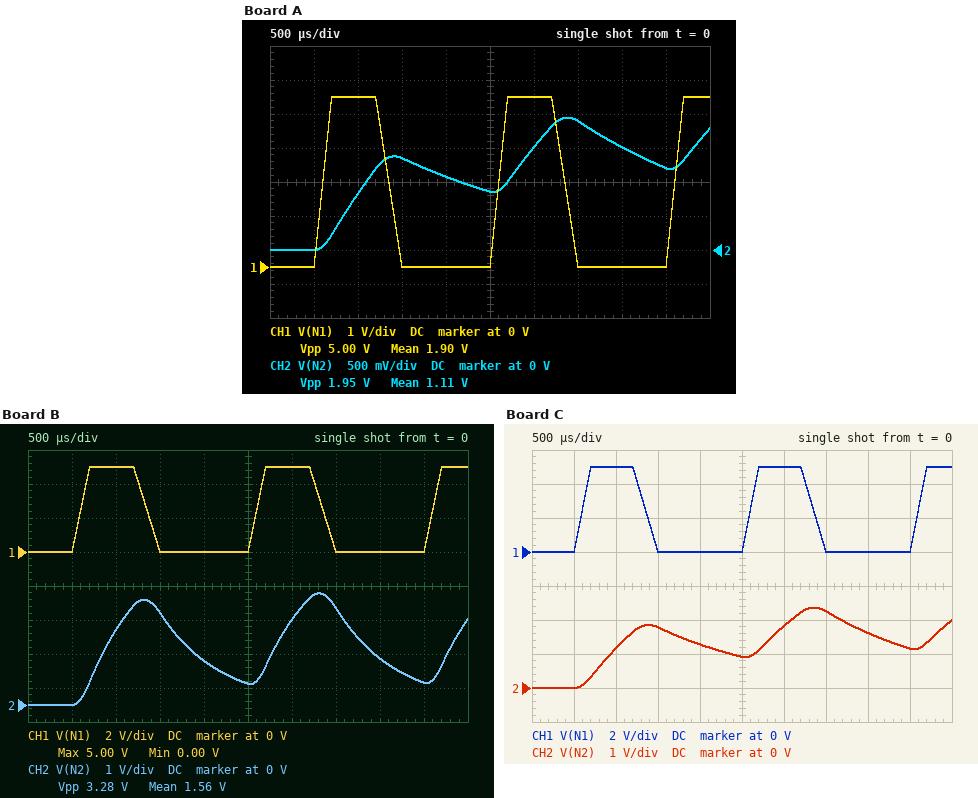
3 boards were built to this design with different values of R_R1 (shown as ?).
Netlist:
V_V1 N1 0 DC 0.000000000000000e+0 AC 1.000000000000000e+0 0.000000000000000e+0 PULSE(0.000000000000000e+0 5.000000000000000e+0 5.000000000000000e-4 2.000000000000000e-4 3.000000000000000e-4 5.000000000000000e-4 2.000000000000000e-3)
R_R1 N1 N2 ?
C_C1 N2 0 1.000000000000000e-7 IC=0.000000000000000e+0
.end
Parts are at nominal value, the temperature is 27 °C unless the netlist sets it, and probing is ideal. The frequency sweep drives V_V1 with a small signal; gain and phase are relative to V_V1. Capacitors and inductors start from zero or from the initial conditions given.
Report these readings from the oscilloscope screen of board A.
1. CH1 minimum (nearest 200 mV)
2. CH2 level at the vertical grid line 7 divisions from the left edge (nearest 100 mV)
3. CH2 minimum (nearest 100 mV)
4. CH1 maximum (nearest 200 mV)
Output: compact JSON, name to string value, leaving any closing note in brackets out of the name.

{"CH1 minimum": "0 V", "CH2 level at the vertical grid line 7 divisions from the left edge": "1.9 V", "CH2 minimum": "0 V", "CH1 maximum": "5.0 V"}
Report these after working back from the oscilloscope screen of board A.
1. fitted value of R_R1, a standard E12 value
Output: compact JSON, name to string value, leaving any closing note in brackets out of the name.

{"fitted value of R_R1, a standard E12 value": "22 kΩ"}
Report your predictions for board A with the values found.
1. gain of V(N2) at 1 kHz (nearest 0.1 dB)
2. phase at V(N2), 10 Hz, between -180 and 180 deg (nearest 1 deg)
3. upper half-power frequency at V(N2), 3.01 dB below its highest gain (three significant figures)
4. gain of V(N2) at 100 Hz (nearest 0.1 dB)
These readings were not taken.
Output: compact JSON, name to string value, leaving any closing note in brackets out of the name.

{"gain of V(N2) at 1 kHz": "-22.8 dB", "phase at V(N2), 10 Hz, between -180 and 180 deg": "-8 deg", "upper half-power frequency at V(N2), 3.01 dB below its highest gain": "72.3 Hz", "gain of V(N2) at 100 Hz": "-4.6 dB"}
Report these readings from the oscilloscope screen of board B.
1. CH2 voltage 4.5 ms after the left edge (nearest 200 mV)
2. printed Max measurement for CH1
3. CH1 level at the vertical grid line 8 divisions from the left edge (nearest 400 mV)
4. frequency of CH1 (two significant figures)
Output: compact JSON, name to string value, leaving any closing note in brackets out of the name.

{"CH2 voltage 4.5 ms after the left edge": "600 mV", "printed Max measurement for CH1": "5.00 V", "CH1 level at the vertical grid line 8 divisions from the left edge": "0 V", "frequency of CH1": "500 Hz"}
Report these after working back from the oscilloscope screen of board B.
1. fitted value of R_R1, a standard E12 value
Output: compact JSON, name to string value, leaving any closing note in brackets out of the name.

{"fitted value of R_R1, a standard E12 value": "6.8 kΩ"}
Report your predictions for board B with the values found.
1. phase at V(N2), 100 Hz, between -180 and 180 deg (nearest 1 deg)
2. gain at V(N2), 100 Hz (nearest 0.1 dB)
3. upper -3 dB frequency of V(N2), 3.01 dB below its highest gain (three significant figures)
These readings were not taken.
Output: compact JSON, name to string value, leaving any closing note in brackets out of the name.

{"phase at V(N2), 100 Hz, between -180 and 180 deg": "-23 deg", "gain at V(N2), 100 Hz": "-0.7 dB", "upper -3 dB frequency of V(N2), 3.01 dB below its highest gain": "234 Hz"}
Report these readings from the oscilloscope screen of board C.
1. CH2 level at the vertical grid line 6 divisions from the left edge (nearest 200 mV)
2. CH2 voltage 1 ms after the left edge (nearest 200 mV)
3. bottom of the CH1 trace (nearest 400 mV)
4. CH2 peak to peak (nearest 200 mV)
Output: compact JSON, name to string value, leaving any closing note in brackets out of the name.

{"CH2 level at the vertical grid line 6 divisions from the left edge": "1.8 V", "CH2 voltage 1 ms after the left edge": "1.2 V", "bottom of the CH1 trace": "0 V", "CH2 peak to peak": "2.4 V"}
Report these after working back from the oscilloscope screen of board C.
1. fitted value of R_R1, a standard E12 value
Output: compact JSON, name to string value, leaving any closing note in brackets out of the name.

{"fitted value of R_R1, a standard E12 value": "15 kΩ"}
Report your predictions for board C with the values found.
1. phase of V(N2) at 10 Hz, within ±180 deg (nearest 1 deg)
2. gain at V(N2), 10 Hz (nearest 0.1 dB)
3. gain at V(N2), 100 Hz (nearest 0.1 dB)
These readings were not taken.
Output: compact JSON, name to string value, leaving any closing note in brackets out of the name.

{"phase of V(N2) at 10 Hz, within ±180 deg": "-5 deg", "gain at V(N2), 10 Hz": "0 dB", "gain at V(N2), 100 Hz": "-2.8 dB"}
